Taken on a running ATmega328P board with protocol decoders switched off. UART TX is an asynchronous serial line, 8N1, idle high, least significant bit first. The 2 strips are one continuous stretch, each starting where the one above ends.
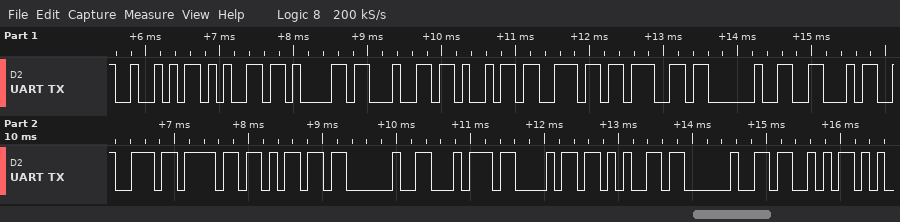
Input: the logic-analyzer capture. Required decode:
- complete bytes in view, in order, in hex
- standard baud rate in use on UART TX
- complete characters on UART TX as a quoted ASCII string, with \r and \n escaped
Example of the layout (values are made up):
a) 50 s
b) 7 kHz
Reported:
a) 52 65 61 64 69 6E 67 20 46 72 6F 6D 20 74 68 65 20 53
b) 9600 baud
c) "Reading From the S"
